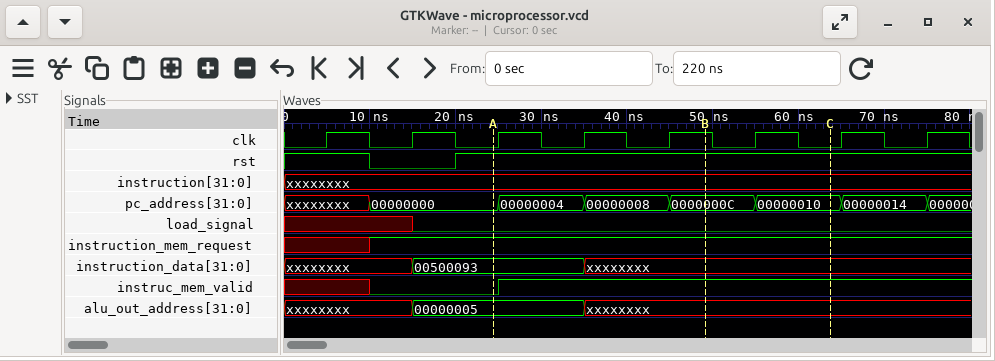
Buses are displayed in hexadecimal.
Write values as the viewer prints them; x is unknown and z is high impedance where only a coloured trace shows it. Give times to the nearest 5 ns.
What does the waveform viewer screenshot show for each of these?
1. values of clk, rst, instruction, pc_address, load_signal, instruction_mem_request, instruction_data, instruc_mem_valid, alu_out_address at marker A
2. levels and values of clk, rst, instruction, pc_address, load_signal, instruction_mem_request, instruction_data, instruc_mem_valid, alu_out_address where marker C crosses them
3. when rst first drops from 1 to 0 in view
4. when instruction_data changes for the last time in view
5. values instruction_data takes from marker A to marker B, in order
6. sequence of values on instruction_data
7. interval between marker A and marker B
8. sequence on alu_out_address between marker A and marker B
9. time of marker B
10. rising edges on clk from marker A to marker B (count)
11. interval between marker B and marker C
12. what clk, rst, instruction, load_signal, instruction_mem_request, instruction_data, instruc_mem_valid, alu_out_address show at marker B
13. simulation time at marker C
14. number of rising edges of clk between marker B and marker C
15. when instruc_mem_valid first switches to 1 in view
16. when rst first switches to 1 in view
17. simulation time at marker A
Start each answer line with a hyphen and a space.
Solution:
- clk=0, rst=1, instruction=xxxxxxxx, pc_address=00000000, load_signal=0, instruction_mem_request=1, instruction_data=00500093, instruc_mem_valid=0, alu_out_address=00000005
- clk=0, rst=1, instruction=xxxxxxxx, pc_address=00000010, load_signal=0, instruction_mem_request=1, instruction_data=xxxxxxxx, instruc_mem_valid=1, alu_out_address=xxxxxxxx
- 10 ns
- 35 ns
- 00500093, xxxxxxxx
- xxxxxxxx, 00500093, xxxxxxxx
- 25 ns
- 00000005, xxxxxxxx
- 50 ns
- 3
- 15 ns
- clk=1, rst=1, instruction=xxxxxxxx, load_signal=0, instruction_mem_request=1, instruction_data=xxxxxxxx, instruc_mem_valid=1, alu_out_address=xxxxxxxx
- 65 ns
- 1
- 25 ns
- 20 ns
- 25 ns
